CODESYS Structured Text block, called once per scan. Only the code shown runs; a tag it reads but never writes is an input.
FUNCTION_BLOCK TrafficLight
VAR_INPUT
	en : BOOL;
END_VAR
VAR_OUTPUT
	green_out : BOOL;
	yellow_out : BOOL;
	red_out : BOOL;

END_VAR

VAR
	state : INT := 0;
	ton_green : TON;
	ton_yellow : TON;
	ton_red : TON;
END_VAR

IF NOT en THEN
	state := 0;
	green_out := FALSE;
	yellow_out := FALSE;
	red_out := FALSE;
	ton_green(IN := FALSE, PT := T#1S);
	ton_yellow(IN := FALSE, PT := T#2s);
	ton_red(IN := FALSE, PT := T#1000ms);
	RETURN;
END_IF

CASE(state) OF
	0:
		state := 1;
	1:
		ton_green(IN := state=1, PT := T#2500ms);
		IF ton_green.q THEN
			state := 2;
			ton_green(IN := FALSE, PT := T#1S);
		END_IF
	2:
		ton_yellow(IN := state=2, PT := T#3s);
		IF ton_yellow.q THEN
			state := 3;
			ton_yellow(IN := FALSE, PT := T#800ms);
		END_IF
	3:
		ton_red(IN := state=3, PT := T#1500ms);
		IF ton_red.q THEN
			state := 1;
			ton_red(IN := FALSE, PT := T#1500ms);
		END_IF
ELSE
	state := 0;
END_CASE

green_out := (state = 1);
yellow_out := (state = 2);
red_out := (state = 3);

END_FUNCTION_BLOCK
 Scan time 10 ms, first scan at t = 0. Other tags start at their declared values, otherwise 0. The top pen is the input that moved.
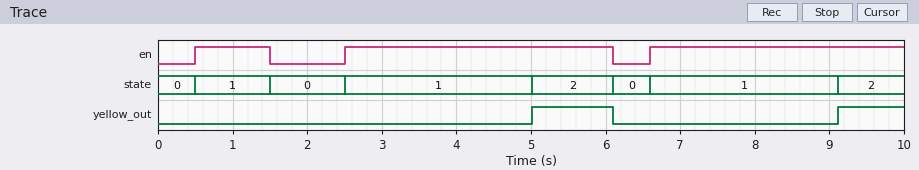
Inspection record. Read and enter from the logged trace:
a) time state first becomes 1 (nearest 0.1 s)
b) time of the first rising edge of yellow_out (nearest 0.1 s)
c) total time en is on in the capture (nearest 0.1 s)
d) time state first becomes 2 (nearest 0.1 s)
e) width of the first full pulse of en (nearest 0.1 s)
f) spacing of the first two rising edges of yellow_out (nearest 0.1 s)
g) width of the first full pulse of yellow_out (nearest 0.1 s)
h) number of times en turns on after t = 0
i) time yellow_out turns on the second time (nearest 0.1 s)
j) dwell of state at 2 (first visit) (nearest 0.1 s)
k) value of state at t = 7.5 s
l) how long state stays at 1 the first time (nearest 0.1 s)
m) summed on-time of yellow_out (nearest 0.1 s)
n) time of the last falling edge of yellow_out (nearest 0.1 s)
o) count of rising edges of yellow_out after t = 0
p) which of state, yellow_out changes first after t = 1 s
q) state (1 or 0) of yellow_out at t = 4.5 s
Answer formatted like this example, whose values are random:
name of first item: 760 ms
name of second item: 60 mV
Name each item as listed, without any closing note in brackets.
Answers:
time state first becomes 1: 0.5 s
time of the first rising edge of yellow_out: 5.0 s
total time en is on in the capture: 8.0 s
time state first becomes 2: 5.0 s
width of the first full pulse of en: 1.0 s
spacing of the first two rising edges of yellow_out: 4.1 s
width of the first full pulse of yellow_out: 1.1 s
number of times en turns on after t = 0: 3
time yellow_out turns on the second time: 9.1 s
dwell of state at 2 (first visit): 1.1 s
value of state at t = 7.5 s: 1
how long state stays at 1 the first time: 1.0 s
summed on-time of yellow_out: 2.0 s
time of the last falling edge of yellow_out: 6.1 s
count of rising edges of yellow_out after t = 0: 2
which of state, yellow_out changes first after t = 1 s: state
state (1 or 0) of yellow_out at t = 4.5 s: 0
